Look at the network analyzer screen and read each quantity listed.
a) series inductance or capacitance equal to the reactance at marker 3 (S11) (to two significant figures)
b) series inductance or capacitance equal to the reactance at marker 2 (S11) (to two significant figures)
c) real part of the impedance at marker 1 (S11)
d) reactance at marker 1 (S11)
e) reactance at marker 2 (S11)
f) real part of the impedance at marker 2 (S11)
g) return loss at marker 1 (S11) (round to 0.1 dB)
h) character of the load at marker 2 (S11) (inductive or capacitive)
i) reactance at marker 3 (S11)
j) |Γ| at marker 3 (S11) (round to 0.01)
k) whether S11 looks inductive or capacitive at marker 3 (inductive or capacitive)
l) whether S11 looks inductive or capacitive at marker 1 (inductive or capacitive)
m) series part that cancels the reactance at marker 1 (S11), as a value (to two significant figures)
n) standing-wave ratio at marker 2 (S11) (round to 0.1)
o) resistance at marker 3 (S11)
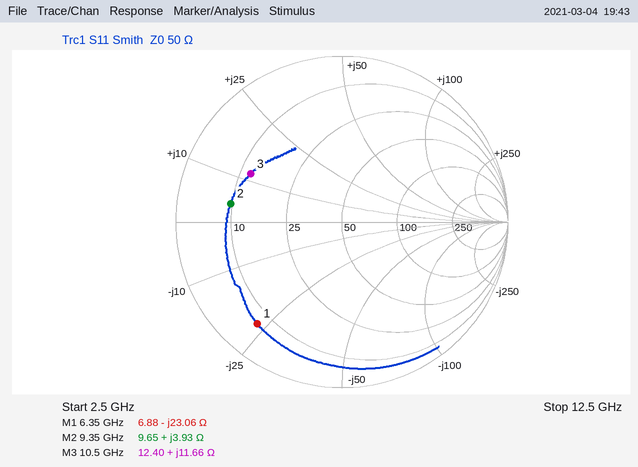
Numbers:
180 pH
67 pH
6.88 Ω
-23.06 Ω
+3.93 Ω
9.65 Ω
2.0 dB
inductive
+11.66 Ω
0.62
inductive
capacitive
580 pH
5.2
12.40 Ω
